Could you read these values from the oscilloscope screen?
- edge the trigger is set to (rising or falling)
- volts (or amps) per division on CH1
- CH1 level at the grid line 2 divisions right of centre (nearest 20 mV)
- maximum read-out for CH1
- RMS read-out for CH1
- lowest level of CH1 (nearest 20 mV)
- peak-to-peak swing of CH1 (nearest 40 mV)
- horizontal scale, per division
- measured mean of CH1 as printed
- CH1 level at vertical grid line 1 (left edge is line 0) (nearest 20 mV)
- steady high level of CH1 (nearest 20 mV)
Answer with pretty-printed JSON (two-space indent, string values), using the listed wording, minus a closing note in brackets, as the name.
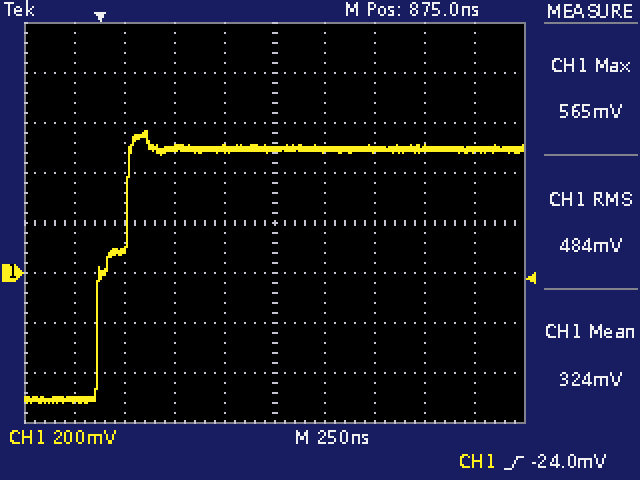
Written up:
{
  "edge the trigger is set to": "rising",
  "volts (or amps) per division on CH1": "200 mV",
  "CH1 level at the grid line 2 divisions right of centre": "500 mV",
  "maximum read-out for CH1": "565 mV",
  "RMS read-out for CH1": "484 mV",
  "lowest level of CH1": "-520 mV",
  "peak-to-peak swing of CH1": "1.08 V",
  "horizontal scale, per division": "250 ns",
  "measured mean of CH1 as printed": "324 mV",
  "CH1 level at vertical grid line 1 (left edge is line 0)": "-500 mV",
  "steady high level of CH1": "500 mV"
}
